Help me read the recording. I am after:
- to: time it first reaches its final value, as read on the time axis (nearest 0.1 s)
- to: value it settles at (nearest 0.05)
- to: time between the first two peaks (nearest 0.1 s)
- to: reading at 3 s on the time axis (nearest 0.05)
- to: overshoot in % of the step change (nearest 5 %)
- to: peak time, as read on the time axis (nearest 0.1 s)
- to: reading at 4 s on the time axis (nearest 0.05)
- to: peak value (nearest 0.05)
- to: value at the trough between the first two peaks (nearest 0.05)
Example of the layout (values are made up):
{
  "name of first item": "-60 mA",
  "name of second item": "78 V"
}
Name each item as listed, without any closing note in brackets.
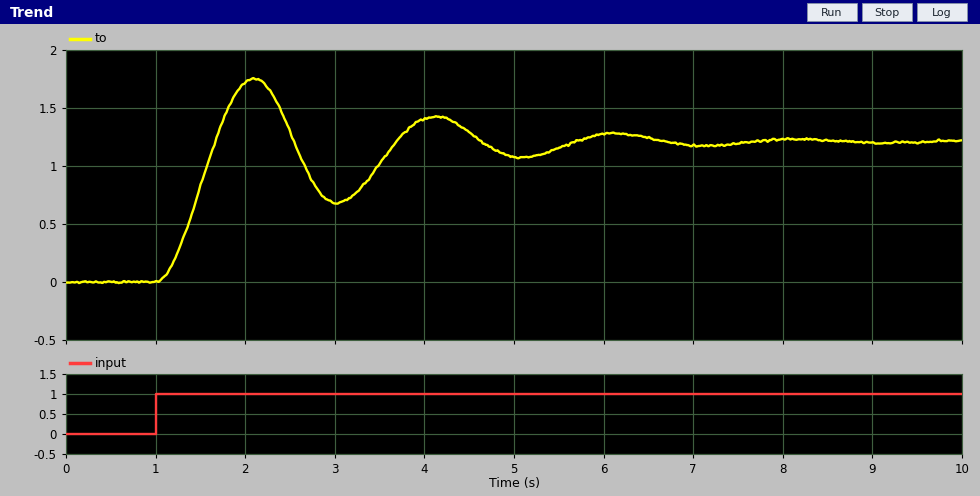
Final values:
{
  "to: time it first reaches its final value, as read on the time axis": "1.7 s",
  "to: value it settles at": "1.20",
  "to: time between the first two peaks": "2.0 s",
  "to: reading at 3 s on the time axis": "0.70",
  "to: overshoot in % of the step change": "45 %",
  "to: peak time, as read on the time axis": "2.1 s",
  "to: reading at 4 s on the time axis": "1.40",
  "to: peak value": "1.75",
  "to: value at the trough between the first two peaks": "0.70"
}
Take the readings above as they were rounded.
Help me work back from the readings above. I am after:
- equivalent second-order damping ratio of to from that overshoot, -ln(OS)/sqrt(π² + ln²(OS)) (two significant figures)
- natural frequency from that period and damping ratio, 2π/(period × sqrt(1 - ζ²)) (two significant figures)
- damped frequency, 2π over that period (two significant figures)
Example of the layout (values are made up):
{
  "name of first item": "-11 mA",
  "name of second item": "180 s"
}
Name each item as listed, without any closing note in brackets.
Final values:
{
  "equivalent second-order damping ratio of to from that overshoot, -ln(OS)/sqrt(π² + ln²(OS))": "0.25",
  "natural frequency from that period and damping ratio, 2π/(period × sqrt(1 - ζ²))": "3.2 rad/s",
  "damped frequency, 2π over that period": "3.1 rad/s"
}
